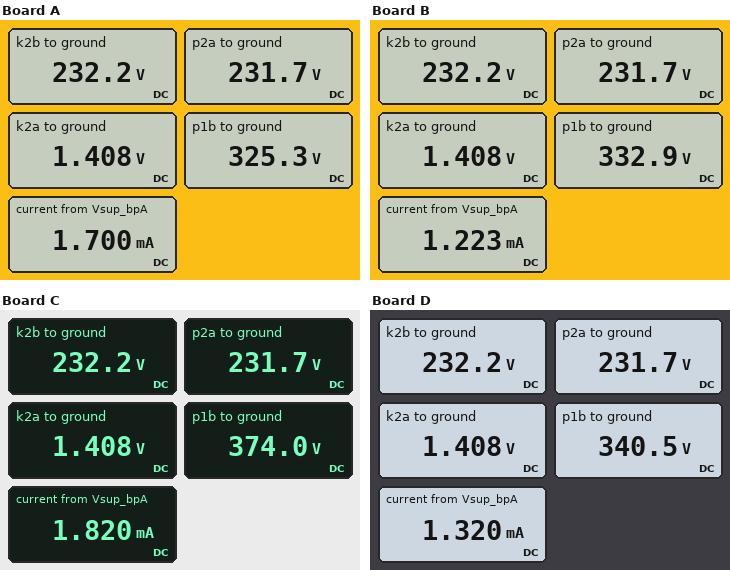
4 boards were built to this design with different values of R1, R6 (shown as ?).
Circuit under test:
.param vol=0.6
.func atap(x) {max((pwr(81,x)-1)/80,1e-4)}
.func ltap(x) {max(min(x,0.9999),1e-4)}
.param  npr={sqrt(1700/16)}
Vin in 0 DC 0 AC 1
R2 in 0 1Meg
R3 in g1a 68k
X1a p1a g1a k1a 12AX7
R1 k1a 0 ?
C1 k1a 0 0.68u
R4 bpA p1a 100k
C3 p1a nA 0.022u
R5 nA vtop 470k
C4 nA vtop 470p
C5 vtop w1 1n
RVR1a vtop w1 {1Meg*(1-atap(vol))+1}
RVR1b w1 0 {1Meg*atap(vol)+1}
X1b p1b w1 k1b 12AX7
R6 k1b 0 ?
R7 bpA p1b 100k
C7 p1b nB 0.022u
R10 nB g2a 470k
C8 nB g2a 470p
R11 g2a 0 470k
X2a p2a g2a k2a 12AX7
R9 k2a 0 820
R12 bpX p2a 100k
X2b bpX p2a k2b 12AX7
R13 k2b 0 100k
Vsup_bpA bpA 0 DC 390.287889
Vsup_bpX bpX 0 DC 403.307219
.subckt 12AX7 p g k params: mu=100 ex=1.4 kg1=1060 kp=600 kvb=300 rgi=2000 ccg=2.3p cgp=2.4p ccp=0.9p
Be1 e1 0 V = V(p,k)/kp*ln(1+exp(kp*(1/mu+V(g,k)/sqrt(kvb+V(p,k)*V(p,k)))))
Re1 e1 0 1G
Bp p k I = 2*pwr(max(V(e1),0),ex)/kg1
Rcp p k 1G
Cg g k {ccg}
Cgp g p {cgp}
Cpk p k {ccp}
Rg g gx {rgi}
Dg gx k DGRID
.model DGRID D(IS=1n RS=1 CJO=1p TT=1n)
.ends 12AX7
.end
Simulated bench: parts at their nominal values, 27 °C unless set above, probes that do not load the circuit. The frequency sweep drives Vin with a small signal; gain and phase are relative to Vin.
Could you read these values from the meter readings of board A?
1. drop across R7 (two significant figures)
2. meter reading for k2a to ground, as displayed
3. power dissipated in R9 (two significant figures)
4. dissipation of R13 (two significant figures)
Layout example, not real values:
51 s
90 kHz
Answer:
65 V
1.408 V
2.4 mW
540 mW
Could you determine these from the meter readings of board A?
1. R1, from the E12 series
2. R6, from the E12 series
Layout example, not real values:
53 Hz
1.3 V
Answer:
2.2 kΩ
4.7 kΩ
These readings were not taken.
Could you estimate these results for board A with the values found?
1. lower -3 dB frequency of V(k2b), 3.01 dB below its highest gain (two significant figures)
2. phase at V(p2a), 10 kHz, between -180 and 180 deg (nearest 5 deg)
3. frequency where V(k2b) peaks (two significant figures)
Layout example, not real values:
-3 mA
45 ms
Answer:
2.2 kHz
145 deg
6.2 kHz
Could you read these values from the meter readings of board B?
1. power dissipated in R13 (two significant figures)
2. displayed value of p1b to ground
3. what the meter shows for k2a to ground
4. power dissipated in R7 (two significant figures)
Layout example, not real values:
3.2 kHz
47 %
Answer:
540 mW
332.9 V
1.408 V
33 mW
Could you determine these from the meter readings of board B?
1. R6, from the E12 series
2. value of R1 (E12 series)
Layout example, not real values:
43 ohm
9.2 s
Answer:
5.6 kΩ
4.7 kΩ
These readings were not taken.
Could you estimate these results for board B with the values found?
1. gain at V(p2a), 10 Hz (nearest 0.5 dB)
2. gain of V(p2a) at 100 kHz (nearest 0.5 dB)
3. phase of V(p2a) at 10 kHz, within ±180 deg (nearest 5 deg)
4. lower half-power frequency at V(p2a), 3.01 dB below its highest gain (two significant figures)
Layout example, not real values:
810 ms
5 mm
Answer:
49.0 dB
57.5 dB
150 deg
2.2 kHz
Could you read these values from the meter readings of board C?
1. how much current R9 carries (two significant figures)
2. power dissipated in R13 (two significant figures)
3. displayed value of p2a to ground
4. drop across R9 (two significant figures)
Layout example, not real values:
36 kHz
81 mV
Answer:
1.7 mA
540 mW
231.7 V
1.4 V
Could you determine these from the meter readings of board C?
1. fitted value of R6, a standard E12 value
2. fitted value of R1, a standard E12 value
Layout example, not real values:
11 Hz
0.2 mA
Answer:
27 kΩ
820 Ω
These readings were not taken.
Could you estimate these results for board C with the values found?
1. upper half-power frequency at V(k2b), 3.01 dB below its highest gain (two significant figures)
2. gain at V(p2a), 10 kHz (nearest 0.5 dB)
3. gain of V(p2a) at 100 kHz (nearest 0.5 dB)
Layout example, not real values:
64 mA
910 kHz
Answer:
16 kHz
71.5 dB
45.0 dB
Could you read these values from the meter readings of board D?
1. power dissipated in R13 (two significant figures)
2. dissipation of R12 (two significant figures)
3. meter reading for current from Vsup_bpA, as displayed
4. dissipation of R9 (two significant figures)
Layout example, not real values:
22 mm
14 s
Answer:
540 mW
290 mW
1.320 mA
2.4 mW
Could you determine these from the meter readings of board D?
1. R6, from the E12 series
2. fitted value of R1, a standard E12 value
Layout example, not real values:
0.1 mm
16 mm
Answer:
6.8 kΩ
3.3 kΩ
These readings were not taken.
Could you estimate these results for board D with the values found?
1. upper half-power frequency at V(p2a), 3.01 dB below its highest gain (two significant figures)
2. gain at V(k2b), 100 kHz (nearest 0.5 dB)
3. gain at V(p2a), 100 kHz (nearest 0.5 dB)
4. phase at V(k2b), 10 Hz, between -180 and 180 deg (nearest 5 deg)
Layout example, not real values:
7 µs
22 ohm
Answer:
17 kHz
56.0 dB
56.0 dB
-115 deg
